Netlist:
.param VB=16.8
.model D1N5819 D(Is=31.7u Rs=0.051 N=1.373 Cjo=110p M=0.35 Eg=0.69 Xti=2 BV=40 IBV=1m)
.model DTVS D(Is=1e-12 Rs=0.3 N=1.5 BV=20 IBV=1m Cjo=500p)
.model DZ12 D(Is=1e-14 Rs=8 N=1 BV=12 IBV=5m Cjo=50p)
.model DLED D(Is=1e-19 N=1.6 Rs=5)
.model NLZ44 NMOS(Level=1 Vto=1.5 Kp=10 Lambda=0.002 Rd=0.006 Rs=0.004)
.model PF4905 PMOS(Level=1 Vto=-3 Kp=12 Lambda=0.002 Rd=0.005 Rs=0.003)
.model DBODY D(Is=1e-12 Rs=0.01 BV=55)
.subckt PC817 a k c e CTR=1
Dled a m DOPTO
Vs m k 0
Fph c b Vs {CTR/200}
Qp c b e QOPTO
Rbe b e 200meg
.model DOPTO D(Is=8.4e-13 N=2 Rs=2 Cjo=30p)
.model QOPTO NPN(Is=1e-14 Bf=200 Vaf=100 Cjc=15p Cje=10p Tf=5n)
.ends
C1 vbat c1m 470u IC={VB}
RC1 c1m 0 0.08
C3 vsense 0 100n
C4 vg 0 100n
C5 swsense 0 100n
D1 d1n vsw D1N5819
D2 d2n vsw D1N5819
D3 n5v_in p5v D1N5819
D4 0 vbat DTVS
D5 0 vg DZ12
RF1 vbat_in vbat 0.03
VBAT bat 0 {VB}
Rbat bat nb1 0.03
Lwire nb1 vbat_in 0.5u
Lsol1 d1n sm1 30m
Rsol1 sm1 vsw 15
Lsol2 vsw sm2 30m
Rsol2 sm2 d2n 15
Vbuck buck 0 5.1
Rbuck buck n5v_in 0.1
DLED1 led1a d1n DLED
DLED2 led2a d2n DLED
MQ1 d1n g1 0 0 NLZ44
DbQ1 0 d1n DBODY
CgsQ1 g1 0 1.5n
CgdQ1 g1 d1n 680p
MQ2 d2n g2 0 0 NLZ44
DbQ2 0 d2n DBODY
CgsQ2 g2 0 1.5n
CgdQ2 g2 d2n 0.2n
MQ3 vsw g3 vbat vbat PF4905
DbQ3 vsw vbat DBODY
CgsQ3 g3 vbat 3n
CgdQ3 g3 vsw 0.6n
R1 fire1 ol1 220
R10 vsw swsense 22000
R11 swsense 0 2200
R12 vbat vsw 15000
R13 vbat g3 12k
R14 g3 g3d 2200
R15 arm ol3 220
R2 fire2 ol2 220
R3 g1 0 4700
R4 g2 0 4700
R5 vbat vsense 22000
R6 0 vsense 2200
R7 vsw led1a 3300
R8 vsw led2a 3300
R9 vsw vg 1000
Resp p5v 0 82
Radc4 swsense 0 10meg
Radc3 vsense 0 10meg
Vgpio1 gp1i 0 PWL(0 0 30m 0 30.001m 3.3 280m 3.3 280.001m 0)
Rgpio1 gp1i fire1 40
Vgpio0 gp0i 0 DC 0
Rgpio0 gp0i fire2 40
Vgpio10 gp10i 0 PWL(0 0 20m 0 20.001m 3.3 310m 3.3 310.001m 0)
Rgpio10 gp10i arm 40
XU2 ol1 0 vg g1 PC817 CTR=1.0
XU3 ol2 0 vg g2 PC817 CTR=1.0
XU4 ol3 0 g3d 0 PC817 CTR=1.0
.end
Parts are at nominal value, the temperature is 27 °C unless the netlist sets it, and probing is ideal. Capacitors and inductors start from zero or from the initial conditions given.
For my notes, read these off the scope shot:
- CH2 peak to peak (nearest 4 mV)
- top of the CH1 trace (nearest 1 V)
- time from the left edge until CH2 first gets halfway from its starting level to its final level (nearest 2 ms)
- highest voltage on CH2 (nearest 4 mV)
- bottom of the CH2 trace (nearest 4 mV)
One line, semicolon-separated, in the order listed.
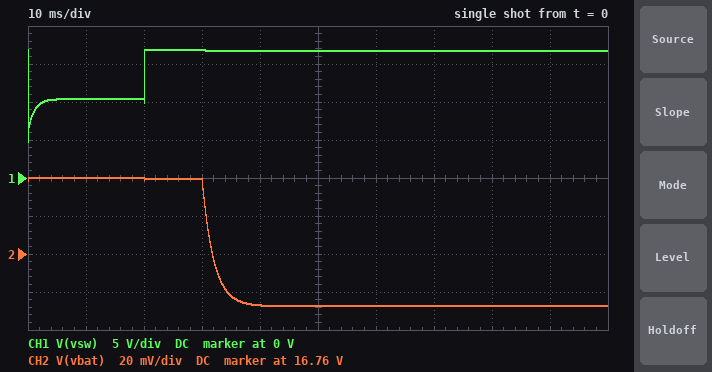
68 mV; 17 V; 32 ms; 16.800 V; 16.732 V
